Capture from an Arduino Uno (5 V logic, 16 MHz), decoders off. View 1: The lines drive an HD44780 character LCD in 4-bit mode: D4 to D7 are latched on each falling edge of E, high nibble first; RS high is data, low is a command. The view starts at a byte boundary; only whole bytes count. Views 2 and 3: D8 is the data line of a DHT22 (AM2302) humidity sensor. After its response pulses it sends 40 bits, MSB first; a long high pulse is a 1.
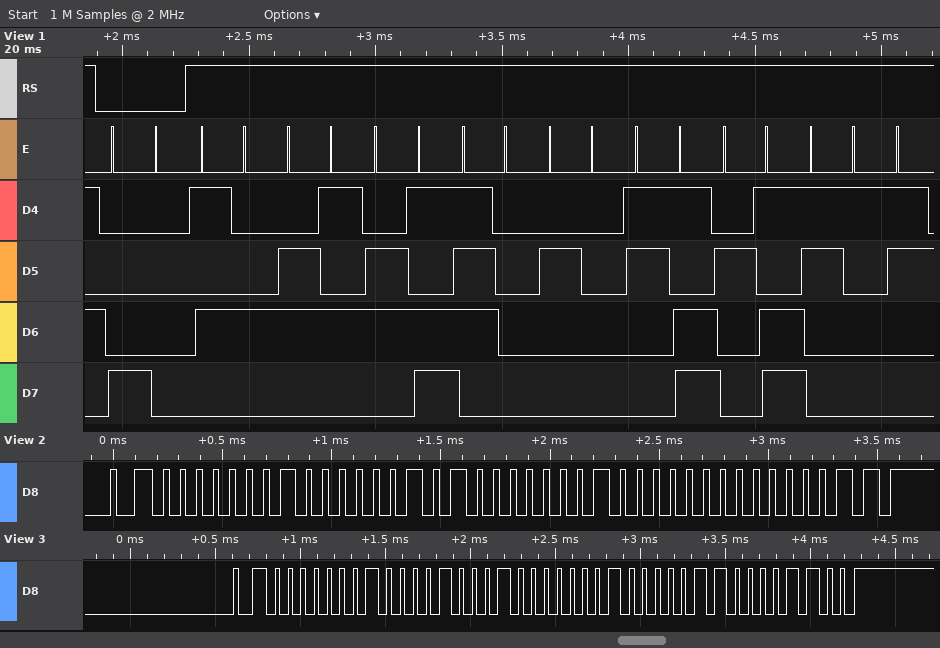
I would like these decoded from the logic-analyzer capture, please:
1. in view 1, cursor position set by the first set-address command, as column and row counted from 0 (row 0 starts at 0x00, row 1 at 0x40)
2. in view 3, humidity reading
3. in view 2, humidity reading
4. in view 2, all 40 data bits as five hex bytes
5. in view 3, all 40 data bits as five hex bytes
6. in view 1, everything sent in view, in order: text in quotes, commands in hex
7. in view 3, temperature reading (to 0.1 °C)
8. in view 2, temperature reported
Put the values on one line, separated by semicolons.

column 0, row 0; 26.4 %; 25.8 %; 01 02 80 80 03; 01 08 80 83 0C; 0x80 "Temp =-1"; -13.1 °C; -12.8 °C
